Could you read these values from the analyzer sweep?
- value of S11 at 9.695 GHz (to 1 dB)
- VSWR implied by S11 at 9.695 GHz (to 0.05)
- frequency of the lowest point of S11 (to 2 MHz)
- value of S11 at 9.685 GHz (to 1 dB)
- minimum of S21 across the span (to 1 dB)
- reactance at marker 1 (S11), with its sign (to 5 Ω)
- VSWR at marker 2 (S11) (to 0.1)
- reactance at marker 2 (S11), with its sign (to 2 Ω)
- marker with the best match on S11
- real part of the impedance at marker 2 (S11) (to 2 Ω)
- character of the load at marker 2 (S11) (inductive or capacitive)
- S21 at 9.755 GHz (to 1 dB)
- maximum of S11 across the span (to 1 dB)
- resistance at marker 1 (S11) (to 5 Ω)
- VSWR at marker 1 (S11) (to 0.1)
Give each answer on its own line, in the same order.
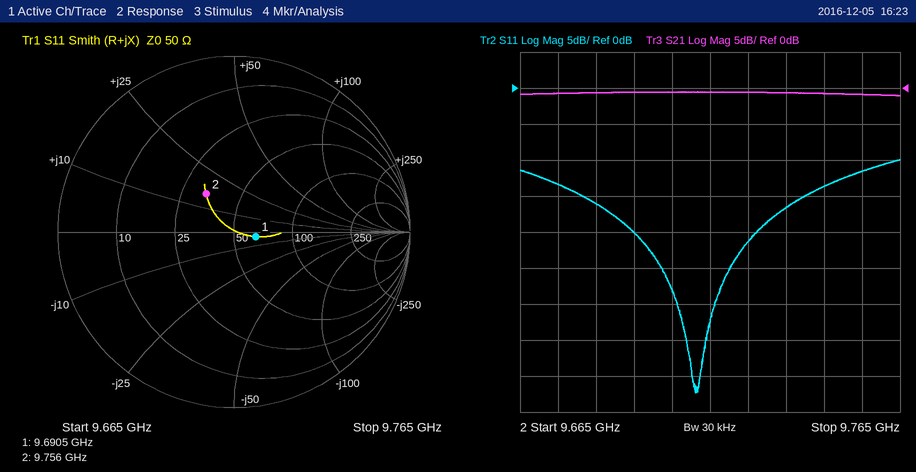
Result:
-20 dB
1.20
9.712 GHz
-16 dB
-1 dB
-5 Ω
1.7
+16 Ω
marker 1
34 Ω
inductive
-1 dB
-10 dB
65 Ω
1.3
